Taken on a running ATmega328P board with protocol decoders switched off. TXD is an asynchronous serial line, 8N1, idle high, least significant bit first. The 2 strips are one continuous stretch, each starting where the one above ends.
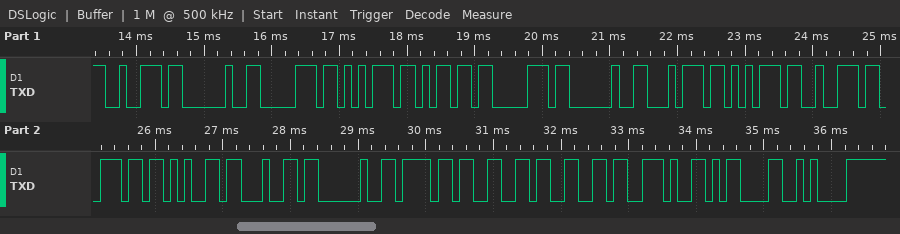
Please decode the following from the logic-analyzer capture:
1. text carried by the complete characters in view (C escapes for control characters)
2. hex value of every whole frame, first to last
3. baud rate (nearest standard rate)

"r pump turned off.\r\n"
72 20 70 75 6D 70 20 74 75 72 6E 65 64 20 6F 66 66 2E 0D 0A
9600 baud
